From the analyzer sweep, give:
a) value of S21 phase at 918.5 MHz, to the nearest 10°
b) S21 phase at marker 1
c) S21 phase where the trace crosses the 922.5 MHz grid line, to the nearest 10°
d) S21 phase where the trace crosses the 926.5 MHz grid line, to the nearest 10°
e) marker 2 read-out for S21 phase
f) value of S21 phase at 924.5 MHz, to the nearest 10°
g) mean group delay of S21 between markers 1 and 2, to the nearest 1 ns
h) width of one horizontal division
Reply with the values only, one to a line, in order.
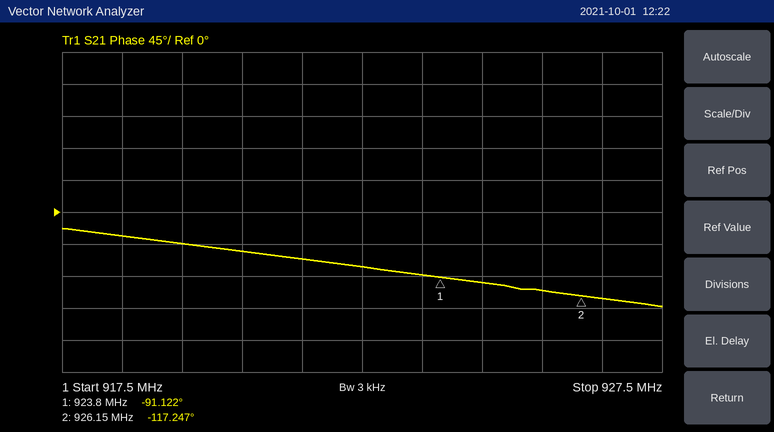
-30°
-91.122°
-80°
-120°
-117.247°
-100°
31 ns
1 MHz
